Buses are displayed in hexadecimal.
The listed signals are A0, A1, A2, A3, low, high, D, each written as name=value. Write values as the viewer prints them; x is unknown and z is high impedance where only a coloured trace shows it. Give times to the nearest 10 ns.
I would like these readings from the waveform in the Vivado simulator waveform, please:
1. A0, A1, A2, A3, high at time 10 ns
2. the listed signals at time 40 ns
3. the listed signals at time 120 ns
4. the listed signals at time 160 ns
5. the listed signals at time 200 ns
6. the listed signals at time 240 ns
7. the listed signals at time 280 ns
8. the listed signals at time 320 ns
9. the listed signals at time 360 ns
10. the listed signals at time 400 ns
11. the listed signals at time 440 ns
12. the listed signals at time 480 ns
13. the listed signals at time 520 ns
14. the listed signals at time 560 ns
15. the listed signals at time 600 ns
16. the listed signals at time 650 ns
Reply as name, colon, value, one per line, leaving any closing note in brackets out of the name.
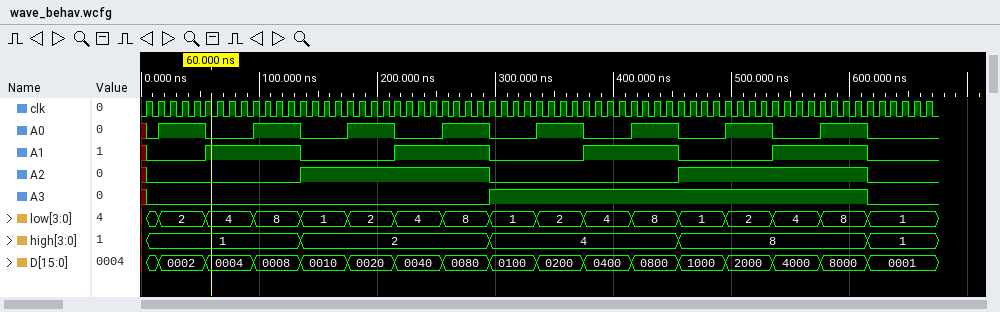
A0, A1, A2, A3, high at time 10 ns: A0=0, A1=0, A2=0, A3=0, high=1
the listed signals at time 40 ns: A0=1, A1=0, A2=0, A3=0, low=2, high=1, D=0002
the listed signals at time 120 ns: A0=1, A1=1, A2=0, A3=0, low=8, high=1, D=0008
the listed signals at time 160 ns: A0=0, A1=0, A2=1, A3=0, low=1, high=2, D=0010
the listed signals at time 200 ns: A0=1, A1=0, A2=1, A3=0, low=2, high=2, D=0020
the listed signals at time 240 ns: A0=0, A1=1, A2=1, A3=0, low=4, high=2, D=0040
the listed signals at time 280 ns: A0=1, A1=1, A2=1, A3=0, low=8, high=2, D=0080
the listed signals at time 320 ns: A0=0, A1=0, A2=0, A3=1, low=1, high=4, D=0100
the listed signals at time 360 ns: A0=1, A1=0, A2=0, A3=1, low=2, high=4, D=0200
the listed signals at time 400 ns: A0=0, A1=1, A2=0, A3=1, low=4, high=4, D=0400
the listed signals at time 440 ns: A0=1, A1=1, A2=0, A3=1, low=8, high=4, D=0800
the listed signals at time 480 ns: A0=0, A1=0, A2=1, A3=1, low=1, high=8, D=1000
the listed signals at time 520 ns: A0=1, A1=0, A2=1, A3=1, low=2, high=8, D=2000
the listed signals at time 560 ns: A0=0, A1=1, A2=1, A3=1, low=4, high=8, D=4000
the listed signals at time 600 ns: A0=1, A1=1, A2=1, A3=1, low=8, high=8, D=8000
the listed signals at time 650 ns: A0=0, A1=0, A2=0, A3=0, low=1, high=1, D=0001
